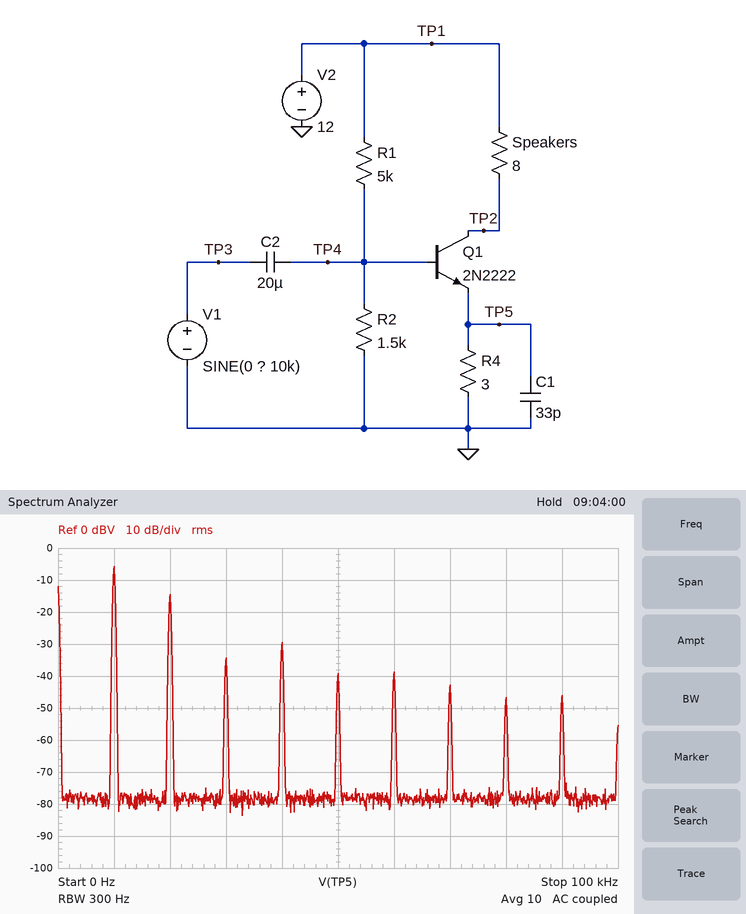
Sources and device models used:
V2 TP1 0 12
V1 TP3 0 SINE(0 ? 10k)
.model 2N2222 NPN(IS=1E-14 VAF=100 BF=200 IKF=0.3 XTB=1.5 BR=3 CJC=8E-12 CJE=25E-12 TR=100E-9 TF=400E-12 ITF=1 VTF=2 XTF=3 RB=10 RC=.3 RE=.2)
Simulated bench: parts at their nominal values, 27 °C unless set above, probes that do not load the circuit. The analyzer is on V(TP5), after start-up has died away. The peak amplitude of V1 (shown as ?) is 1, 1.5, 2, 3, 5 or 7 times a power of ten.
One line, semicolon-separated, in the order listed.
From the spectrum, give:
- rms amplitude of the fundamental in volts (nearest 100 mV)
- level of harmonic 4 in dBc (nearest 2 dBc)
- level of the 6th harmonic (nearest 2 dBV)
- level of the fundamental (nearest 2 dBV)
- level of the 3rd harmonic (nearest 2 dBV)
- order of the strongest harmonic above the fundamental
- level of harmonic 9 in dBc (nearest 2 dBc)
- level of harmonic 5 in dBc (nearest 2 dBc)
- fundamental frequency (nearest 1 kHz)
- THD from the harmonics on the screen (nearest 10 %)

500 mV; -24 dBc; -38 dBV; -6 dBV; -34 dBV; 2; -40 dBc; -34 dBc; 10 kHz; 40 %
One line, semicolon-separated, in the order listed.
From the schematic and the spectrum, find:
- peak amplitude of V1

1.5 V
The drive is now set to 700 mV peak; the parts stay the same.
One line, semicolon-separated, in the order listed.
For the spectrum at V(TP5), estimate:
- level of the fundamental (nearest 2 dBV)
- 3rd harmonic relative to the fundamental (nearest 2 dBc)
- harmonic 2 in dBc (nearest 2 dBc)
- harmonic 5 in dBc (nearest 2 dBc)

-8 dBV; -28 dBc; -22 dBc; -40 dBc
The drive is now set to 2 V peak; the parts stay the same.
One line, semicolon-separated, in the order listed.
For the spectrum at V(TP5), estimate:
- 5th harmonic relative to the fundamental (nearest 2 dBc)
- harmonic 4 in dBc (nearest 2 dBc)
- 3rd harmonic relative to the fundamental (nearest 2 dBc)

-38 dBc; -22 dBc; -32 dBc
